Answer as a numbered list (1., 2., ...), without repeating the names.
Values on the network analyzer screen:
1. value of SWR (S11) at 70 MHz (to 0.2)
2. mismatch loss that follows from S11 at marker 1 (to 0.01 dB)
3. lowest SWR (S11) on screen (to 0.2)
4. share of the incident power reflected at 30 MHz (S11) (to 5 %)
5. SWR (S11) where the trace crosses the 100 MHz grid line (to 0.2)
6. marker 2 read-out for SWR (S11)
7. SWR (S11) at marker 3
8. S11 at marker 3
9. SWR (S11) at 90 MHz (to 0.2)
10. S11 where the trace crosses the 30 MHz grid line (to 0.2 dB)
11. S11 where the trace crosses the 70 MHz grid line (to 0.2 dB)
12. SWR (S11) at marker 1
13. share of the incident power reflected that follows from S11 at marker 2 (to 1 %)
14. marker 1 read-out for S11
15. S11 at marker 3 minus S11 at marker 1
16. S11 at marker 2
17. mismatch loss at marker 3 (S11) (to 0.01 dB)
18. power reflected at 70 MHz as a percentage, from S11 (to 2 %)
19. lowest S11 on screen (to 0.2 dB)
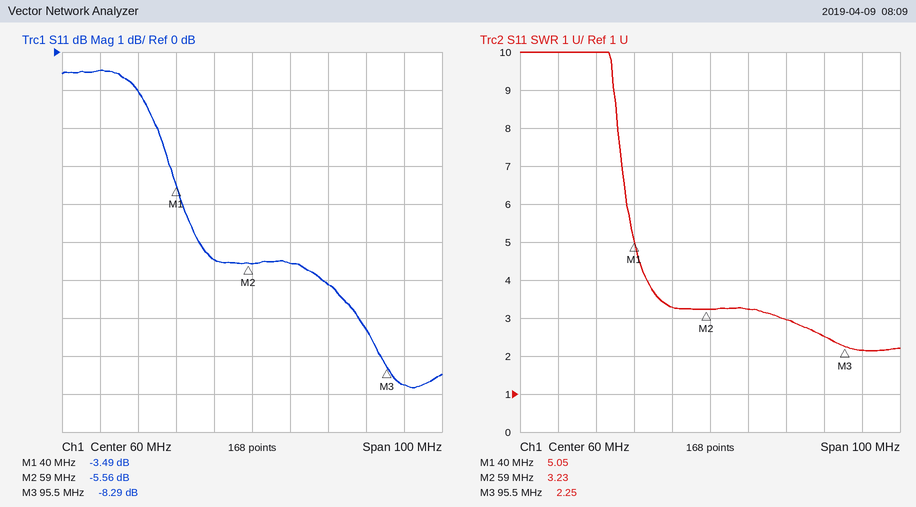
1. 3.2
2. 2.58 dB
3. 2.2
4. 80 %
5. 2.2
6. 3.23
7. 2.25
8. -8.29 dB
9. 2.6
10. -1.0 dB
11. -5.6 dB
12. 5.05
13. 28 %
14. -3.49 dB
15. -4.80 dB
16. -5.56 dB
17. 0.70 dB
18. 28 %
19. -8.8 dB
